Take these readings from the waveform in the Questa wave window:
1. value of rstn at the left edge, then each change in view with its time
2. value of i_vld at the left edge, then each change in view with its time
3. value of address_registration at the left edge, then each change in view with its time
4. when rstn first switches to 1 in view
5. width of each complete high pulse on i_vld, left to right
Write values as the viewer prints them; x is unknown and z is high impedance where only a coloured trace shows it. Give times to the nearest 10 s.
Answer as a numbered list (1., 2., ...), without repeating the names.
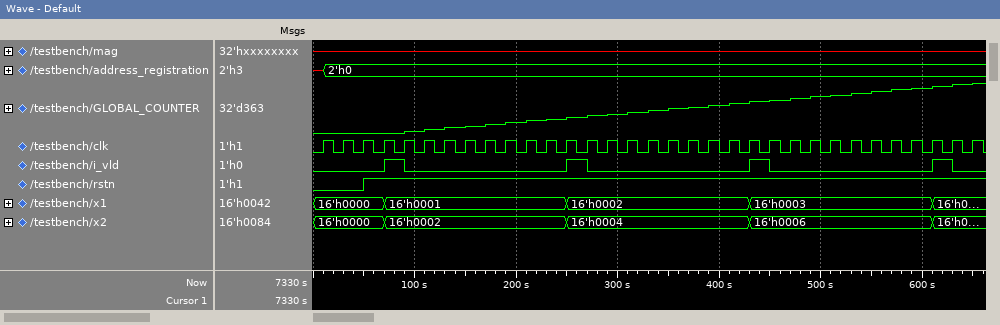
1. 0, 1 at 50 s
2. 0, 1 at 70 s, 0 at 90 s, 1 at 250 s, 0 at 270 s, 1 at 430 s, 0 at 450 s, 1 at 610 s, 0 at 630 s
3. x, 2'h0 at 10 s
4. 50 s
5. 20 s, 20 s, 20 s, 20 s
